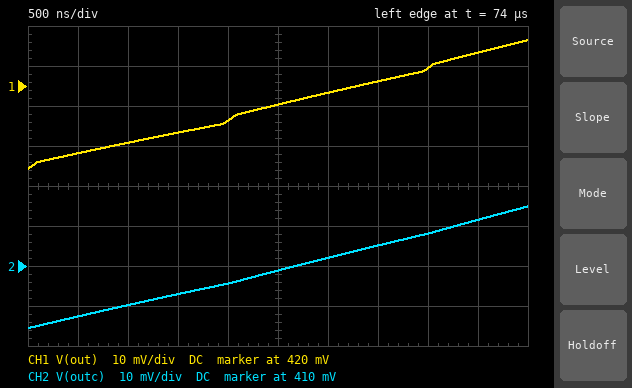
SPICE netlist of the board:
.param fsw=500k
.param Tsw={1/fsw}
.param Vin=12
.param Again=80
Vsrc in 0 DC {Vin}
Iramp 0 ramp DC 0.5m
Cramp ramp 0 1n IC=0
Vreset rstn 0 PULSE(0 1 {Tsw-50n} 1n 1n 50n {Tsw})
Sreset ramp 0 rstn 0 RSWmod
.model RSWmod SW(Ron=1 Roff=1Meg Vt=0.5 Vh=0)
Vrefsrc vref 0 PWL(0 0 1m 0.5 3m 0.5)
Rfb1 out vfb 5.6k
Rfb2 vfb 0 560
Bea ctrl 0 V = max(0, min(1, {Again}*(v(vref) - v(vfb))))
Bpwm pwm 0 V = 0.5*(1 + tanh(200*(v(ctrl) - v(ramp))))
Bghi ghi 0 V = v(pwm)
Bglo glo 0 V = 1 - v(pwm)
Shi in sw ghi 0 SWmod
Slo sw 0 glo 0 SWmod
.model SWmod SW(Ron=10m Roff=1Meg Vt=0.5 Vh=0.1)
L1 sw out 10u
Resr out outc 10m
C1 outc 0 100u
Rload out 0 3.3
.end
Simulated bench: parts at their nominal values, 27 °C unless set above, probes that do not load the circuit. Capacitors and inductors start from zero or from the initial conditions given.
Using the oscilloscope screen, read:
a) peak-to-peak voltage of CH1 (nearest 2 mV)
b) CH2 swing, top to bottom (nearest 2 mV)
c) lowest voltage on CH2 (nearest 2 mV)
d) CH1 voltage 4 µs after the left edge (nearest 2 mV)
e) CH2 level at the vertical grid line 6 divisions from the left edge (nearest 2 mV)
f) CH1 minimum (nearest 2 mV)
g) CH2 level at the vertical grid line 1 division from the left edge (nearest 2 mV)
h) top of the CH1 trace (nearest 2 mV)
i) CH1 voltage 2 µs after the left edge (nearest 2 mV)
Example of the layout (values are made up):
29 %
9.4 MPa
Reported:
32 mV
30 mV
394 mV
424 mV
412 mV
400 mV
398 mV
432 mV
412 mV
